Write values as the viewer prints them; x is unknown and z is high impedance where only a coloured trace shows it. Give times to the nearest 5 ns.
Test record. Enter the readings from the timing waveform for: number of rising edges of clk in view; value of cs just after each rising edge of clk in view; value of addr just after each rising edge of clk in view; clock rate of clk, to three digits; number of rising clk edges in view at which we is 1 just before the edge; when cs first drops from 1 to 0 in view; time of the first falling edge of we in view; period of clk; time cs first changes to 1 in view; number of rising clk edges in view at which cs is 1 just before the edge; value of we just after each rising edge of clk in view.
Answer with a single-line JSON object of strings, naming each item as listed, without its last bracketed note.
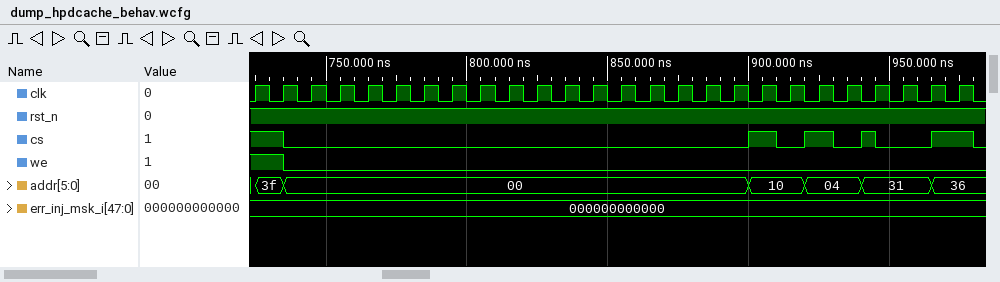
{"number of rising edges of clk in view": "26", "value of cs just after each rising edge of clk in view": "1 0 0 0 0 0 0 0 0 0 0 0 0 0 0 0 0 0 1 0 1 0 0 0 1 1", "value of addr just after each rising edge of clk in view": "3f, 00, 00, 00, 00, 00, 00, 00, 00, 00, 00, 00, 00, 00, 00, 00, 00, 00, 10, 10, 04, 04, 31, 31, 36, 36", "clock rate of clk, to three digits": "100 MHz", "number of rising clk edges in view at which we is 1 just before the edge": "2", "when cs first drops from 1 to 0 in view": "735 ns", "time of the first falling edge of we in view": "735 ns", "period of clk": "10 ns", "time cs first changes to 1 in view": "900 ns", "number of rising clk edges in view at which cs is 1 just before the edge": "6", "value of we just after each rising edge of clk in view": "1 0 0 0 0 0 0 0 0 0 0 0 0 0 0 0 0 0 0 0 0 0 0 0 0 0"}
